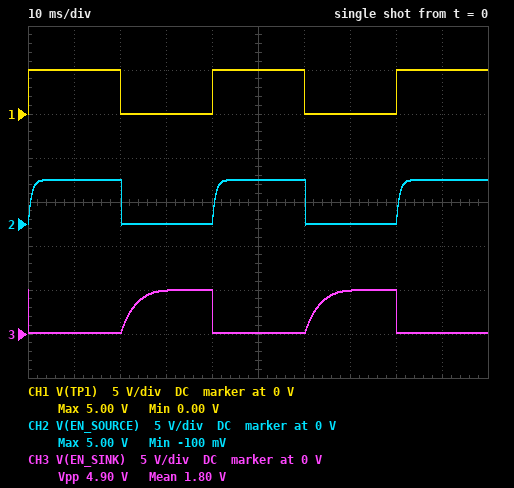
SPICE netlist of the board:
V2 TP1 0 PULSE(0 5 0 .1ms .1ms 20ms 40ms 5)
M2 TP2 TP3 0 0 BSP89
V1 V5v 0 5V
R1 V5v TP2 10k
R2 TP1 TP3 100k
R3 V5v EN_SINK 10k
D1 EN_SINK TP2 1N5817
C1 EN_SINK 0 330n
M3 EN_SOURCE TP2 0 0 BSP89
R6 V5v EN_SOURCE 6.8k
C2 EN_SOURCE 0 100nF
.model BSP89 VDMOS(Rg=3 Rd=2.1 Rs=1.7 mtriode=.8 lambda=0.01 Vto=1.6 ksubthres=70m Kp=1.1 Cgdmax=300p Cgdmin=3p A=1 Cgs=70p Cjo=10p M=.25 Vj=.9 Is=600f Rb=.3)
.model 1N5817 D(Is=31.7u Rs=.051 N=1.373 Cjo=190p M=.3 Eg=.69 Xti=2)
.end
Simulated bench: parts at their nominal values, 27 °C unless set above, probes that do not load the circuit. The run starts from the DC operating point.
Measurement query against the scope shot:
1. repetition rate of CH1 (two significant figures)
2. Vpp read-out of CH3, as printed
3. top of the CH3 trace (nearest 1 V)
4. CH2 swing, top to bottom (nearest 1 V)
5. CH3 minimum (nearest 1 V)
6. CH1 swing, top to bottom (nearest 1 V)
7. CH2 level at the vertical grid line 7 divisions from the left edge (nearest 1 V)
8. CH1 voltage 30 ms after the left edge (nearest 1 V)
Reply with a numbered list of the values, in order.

1. 25 Hz
2. 4.90 V
3. 5 V
4. 5 V
5. 0 V
6. 5 V
7. 0 V
8. 0 V
